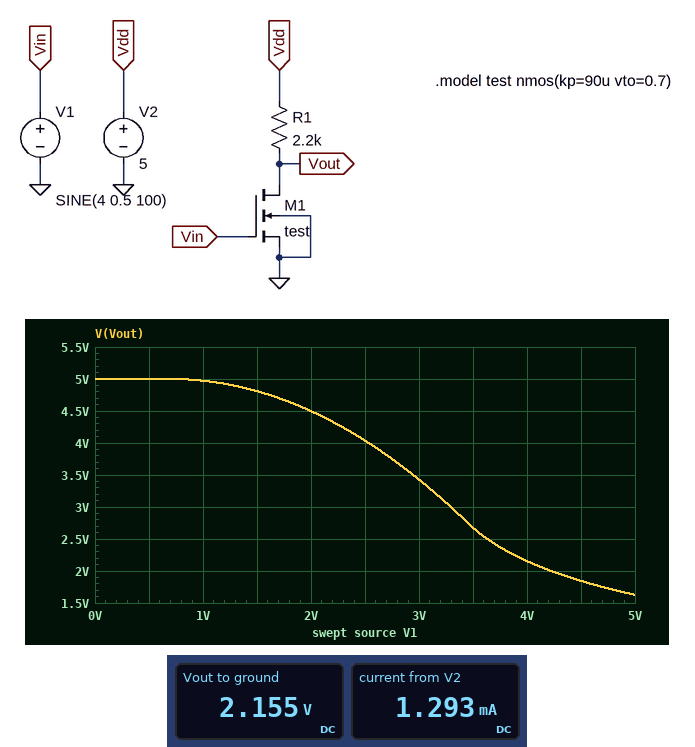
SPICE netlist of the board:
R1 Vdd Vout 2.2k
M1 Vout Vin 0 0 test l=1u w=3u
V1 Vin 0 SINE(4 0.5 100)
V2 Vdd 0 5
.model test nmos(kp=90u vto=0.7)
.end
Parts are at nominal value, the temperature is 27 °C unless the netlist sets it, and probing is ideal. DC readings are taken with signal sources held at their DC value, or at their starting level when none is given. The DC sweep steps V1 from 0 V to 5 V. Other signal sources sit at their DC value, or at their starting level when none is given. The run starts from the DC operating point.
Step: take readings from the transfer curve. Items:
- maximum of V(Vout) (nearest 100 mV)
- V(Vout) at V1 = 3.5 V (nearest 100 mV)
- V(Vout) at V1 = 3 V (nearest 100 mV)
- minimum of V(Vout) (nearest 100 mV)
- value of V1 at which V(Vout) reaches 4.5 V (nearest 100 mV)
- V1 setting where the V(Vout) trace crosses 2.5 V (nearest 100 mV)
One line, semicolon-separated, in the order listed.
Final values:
5.0 V; 2.7 V; 3.4 V; 1.6 V; 2.0 V; 3.6 V
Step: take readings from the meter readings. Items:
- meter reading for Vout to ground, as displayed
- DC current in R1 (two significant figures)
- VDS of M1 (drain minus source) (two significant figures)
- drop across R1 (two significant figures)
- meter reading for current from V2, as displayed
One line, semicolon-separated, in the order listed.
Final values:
2.155 V; 1.3 mA; 2.2 V; 2.8 V; 1.293 mA
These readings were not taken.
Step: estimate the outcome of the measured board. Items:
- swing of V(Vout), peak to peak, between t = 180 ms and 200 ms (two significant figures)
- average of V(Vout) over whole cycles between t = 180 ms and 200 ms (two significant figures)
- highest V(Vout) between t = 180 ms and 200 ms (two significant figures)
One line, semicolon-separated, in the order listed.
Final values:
830 mV; 2.2 V; 2.7 V
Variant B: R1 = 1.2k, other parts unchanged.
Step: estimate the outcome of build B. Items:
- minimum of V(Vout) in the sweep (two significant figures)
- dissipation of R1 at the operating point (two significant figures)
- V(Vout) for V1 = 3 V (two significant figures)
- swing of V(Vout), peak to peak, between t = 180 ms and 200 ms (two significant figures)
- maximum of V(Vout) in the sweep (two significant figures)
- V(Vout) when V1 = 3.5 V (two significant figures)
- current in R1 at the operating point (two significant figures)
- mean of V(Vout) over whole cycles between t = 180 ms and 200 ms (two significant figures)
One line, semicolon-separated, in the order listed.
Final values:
2.5 V; 2.6 mW; 4.1 V; 910 mV; 5.0 V; 3.7 V; 1.5 mA; 3.3 V
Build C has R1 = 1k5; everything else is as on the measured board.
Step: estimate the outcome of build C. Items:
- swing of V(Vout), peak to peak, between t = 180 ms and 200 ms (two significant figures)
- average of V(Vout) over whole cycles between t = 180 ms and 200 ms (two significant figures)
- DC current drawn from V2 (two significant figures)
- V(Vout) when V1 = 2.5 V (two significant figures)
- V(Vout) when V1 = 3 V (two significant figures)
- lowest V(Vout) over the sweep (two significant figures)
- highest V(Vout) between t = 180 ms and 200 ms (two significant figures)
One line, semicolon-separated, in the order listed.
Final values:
970 mV; 2.9 V; 1.4 mA; 4.3 V; 3.9 V; 2.2 V; 3.4 V
